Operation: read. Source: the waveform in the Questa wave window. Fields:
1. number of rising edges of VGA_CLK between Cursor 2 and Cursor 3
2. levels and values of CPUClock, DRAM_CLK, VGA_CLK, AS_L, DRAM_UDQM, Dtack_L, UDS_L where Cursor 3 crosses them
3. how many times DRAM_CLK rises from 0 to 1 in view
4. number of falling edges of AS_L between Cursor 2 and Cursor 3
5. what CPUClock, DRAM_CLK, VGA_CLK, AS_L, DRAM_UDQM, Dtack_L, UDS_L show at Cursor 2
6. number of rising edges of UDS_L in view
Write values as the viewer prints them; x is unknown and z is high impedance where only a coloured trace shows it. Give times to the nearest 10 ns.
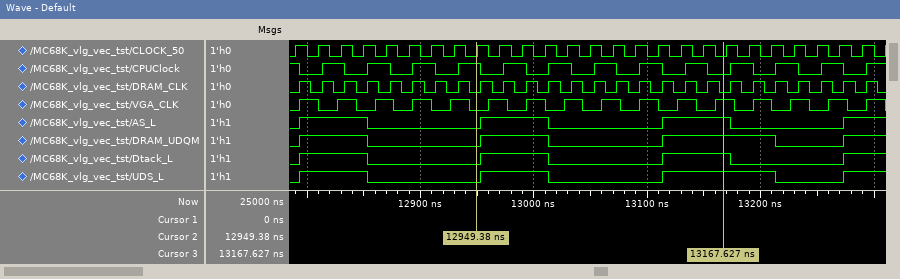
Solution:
7
CPUClock=0, DRAM_CLK=0, VGA_CLK=1, AS_L=1, DRAM_UDQM=1, Dtack_L=1, UDS_L=1
26
1
CPUClock=1, DRAM_CLK=0, VGA_CLK=0, AS_L=0, DRAM_UDQM=0, Dtack_L=0, UDS_L=0
4
